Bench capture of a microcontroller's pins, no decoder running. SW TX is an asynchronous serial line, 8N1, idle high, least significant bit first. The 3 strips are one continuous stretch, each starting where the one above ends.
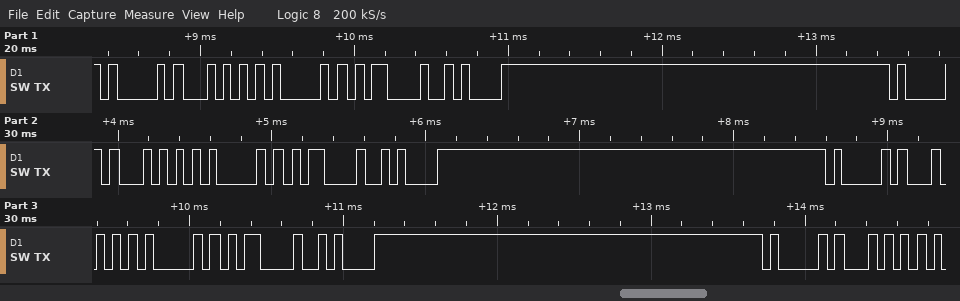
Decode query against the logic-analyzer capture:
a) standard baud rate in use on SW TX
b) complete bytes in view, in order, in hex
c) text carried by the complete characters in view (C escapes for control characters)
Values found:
19200 baud
0x41 0x54 0x41 0x0D 0x0A 0x41 0x54 0x41 0x0D 0x0A 0x41 0x54 0x41 0x0D 0x0A 0x41 0x54
"ATA\r\nATA\r\nATA\r\nAT"
